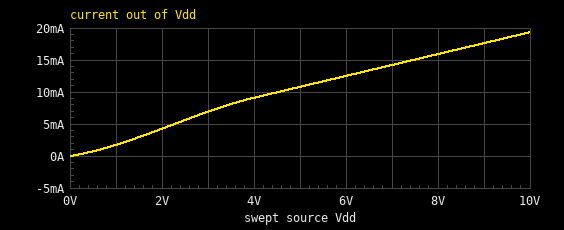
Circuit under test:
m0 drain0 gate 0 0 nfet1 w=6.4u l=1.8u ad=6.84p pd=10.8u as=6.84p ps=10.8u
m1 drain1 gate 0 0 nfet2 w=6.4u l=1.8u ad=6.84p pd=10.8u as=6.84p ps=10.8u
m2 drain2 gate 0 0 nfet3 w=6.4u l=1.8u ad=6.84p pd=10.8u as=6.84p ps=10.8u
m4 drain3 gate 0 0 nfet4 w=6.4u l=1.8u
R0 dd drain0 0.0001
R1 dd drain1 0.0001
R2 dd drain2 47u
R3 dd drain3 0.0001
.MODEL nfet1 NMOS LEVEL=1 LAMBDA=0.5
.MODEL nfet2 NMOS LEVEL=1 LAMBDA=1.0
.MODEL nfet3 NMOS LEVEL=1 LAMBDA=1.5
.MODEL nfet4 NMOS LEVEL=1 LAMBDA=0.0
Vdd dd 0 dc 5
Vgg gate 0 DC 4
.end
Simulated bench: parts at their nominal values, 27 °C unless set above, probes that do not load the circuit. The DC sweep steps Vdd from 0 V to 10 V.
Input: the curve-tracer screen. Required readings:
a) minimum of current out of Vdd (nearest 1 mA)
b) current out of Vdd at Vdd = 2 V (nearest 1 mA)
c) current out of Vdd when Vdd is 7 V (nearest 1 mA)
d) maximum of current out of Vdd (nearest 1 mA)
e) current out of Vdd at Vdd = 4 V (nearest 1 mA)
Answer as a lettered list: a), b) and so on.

a) 0 A
b) 4 mA
c) 14 mA
d) 19 mA
e) 9 mA
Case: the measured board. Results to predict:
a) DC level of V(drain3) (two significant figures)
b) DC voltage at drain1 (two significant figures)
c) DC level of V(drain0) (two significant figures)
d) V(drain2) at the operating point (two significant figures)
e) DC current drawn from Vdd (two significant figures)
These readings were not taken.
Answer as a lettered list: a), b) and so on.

a) 5.0 V
b) 5.0 V
c) 5.0 V
d) 5.0 V
e) 11 mA
